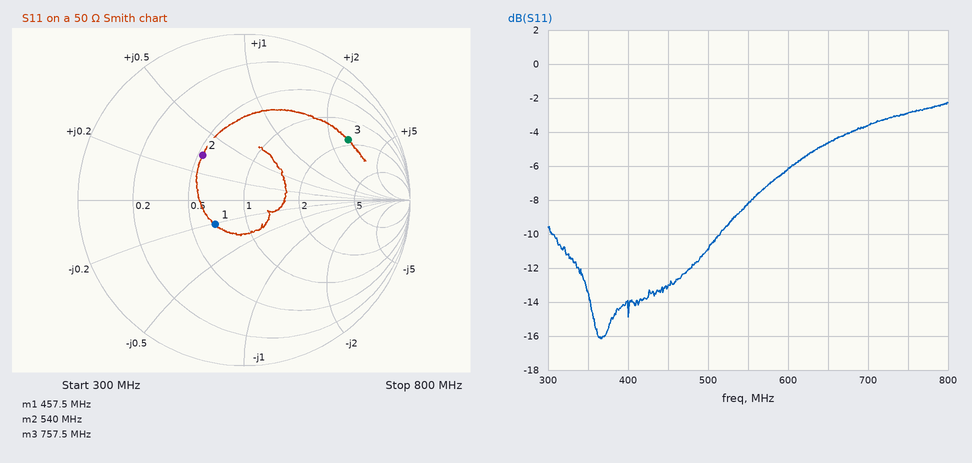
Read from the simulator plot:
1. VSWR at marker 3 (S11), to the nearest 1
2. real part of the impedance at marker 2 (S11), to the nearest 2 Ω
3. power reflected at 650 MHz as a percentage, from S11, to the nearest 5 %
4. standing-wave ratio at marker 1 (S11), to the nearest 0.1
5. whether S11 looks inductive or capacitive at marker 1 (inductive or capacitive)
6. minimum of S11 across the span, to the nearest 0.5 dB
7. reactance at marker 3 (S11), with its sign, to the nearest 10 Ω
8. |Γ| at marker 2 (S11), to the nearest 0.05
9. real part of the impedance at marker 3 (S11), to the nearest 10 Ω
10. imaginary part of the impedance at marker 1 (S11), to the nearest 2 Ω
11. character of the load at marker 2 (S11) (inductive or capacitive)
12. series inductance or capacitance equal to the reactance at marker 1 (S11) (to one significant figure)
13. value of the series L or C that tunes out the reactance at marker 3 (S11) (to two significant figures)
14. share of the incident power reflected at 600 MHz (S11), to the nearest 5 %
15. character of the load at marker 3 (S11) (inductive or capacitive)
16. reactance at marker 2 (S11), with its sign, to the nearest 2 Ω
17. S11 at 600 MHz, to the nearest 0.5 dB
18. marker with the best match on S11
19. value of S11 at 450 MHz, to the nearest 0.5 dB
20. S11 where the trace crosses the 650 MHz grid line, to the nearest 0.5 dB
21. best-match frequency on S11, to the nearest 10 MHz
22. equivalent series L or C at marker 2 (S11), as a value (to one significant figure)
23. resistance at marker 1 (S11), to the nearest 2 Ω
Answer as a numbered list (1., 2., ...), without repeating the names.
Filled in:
1. 6
2. 26 Ω
3. 35 %
4. 1.6
5. capacitive
6. -16.0 dB
7. +130 Ω
8. 0.35
9. 90 Ω
10. -10 Ω
11. inductive
12. 30 pF
13. 1.6 pF
14. 25 %
15. inductive
16. +16 Ω
17. -6.0 dB
18. marker 1
19. -13.0 dB
20. -4.5 dB
21. 370 MHz
22. 5 nH
23. 34 Ω
